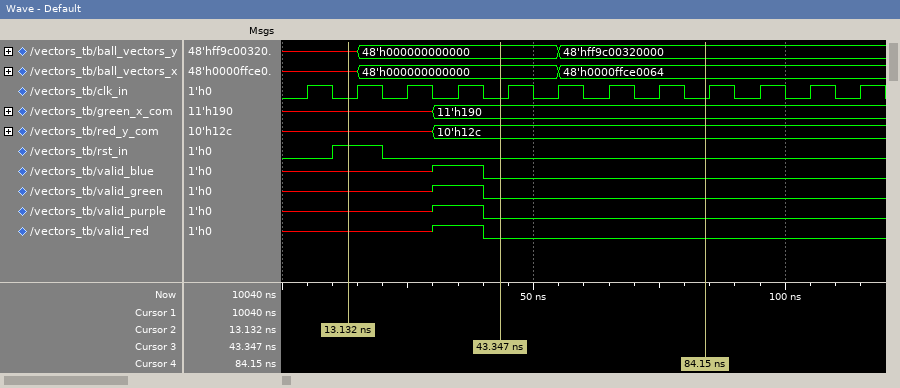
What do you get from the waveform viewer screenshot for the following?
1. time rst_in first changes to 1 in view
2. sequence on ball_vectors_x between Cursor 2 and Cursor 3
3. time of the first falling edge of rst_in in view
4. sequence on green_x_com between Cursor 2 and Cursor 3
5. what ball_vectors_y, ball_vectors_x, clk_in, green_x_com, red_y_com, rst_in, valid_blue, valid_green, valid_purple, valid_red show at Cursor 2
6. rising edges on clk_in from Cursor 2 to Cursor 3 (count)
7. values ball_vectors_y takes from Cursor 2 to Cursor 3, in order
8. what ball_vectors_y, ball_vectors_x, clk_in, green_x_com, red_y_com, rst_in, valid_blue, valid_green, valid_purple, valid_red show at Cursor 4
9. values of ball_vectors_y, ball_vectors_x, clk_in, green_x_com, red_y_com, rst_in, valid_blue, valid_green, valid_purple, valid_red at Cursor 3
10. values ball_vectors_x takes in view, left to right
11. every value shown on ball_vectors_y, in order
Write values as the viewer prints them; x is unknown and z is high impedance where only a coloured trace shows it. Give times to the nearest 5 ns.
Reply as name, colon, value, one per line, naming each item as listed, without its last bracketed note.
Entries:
time rst_in first changes to 1 in view: 10 ns
sequence on ball_vectors_x between Cursor 2 and Cursor 3: x, 48'h000000000000
time of the first falling edge of rst_in in view: 20 ns
sequence on green_x_com between Cursor 2 and Cursor 3: x, 11'h190
what ball_vectors_y, ball_vectors_x, clk_in, green_x_com, red_y_com, rst_in, valid_blue, valid_green, valid_purple, valid_red show at Cursor 2: ball_vectors_y=x, ball_vectors_x=x, clk_in=0, green_x_com=x, red_y_com=x, rst_in=1, valid_blue=x, valid_green=x, valid_purple=x, valid_red=x
rising edges on clk_in from Cursor 2 to Cursor 3: 3
values ball_vectors_y takes from Cursor 2 to Cursor 3, in order: x, 48'h000000000000
what ball_vectors_y, ball_vectors_x, clk_in, green_x_com, red_y_com, rst_in, valid_blue, valid_green, valid_purple, valid_red show at Cursor 4: ball_vectors_y=48'hff9c00320000, ball_vectors_x=48'h0000ffce0064, clk_in=0, green_x_com=11'h190, red_y_com=10'h12c, rst_in=0, valid_blue=0, valid_green=0, valid_purple=0, valid_red=0
values of ball_vectors_y, ball_vectors_x, clk_in, green_x_com, red_y_com, rst_in, valid_blue, valid_green, valid_purple, valid_red at Cursor 3: ball_vectors_y=48'h000000000000, ball_vectors_x=48'h000000000000, clk_in=0, green_x_com=11'h190, red_y_com=10'h12c, rst_in=0, valid_blue=0, valid_green=0, valid_purple=0, valid_red=0
values ball_vectors_x takes in view, left to right: x, 48'h000000000000, 48'h0000ffce0064
every value shown on ball_vectors_y, in order: x, 48'h000000000000, 48'hff9c00320000
